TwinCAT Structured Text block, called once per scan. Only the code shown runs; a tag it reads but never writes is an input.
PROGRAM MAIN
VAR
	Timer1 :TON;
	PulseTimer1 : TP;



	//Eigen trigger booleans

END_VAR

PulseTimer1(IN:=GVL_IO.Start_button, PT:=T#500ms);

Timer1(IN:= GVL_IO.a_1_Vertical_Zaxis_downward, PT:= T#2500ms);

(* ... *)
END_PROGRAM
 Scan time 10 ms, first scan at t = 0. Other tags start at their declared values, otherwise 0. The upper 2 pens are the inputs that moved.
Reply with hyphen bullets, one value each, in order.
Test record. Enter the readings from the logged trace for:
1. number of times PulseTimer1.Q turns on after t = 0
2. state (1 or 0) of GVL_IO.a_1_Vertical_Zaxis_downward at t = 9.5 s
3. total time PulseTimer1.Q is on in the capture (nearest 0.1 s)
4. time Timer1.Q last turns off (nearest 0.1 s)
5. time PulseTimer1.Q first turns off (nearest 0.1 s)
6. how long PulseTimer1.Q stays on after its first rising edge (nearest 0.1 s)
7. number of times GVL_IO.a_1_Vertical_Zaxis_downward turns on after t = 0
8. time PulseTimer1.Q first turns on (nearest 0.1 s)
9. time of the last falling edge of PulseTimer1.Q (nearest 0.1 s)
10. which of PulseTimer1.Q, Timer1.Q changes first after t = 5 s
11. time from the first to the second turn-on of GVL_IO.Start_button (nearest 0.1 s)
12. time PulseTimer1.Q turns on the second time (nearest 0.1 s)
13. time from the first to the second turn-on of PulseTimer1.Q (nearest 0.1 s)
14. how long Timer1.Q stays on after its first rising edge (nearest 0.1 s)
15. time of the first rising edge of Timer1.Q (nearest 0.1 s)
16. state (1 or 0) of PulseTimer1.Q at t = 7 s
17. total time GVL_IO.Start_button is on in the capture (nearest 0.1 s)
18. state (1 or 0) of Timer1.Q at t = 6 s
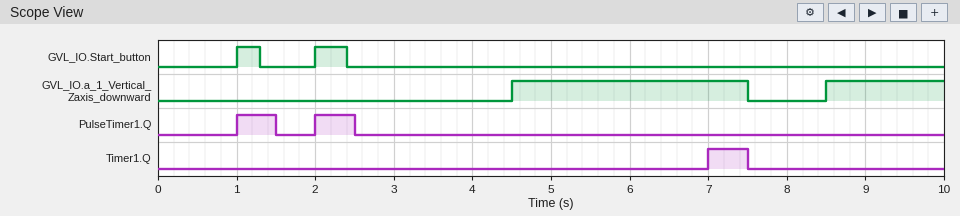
- 2
- 1
- 1.0 s
- 7.5 s
- 1.5 s
- 0.5 s
- 2
- 1.0 s
- 2.5 s
- Timer1.Q
- 1.0 s
- 2.0 s
- 1.0 s
- 0.5 s
- 7.0 s
- 0
- 0.7 s
- 0
